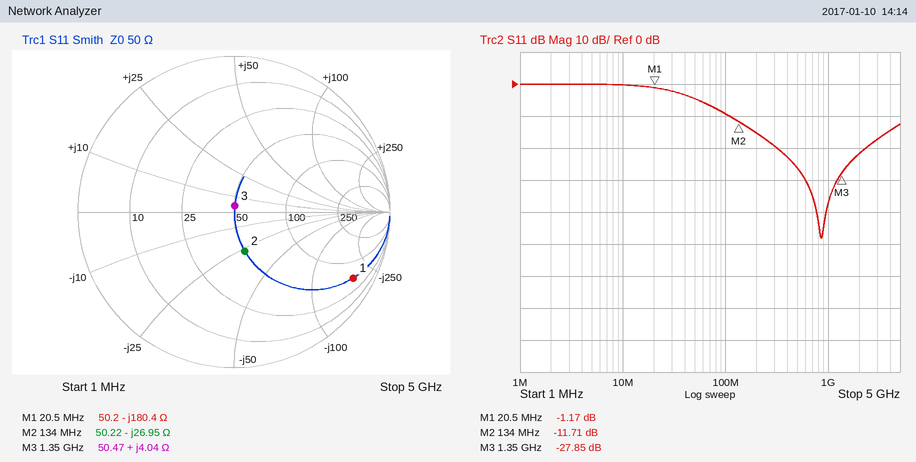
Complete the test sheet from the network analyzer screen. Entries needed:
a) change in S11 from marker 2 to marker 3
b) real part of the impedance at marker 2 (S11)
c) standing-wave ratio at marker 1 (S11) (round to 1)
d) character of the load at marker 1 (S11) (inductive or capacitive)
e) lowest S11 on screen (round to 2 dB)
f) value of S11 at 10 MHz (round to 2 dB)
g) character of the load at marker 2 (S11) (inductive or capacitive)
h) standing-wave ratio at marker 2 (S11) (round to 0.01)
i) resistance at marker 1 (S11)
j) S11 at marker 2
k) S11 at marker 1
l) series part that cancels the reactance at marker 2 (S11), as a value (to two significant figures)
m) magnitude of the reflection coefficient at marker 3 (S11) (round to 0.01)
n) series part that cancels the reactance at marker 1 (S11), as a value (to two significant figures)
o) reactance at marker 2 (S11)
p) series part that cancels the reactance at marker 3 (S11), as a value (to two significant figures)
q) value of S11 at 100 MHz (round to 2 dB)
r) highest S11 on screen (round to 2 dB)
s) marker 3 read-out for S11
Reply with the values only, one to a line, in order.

-16.14 dB
50.22 Ω
15
capacitive
-48 dB
0 dB
capacitive
1.70
50.2 Ω
-11.71 dB
-1.17 dB
32 nH
0.04
1.4 µH
-26.95 Ω
29 pF
-10 dB
0 dB
-27.85 dB
